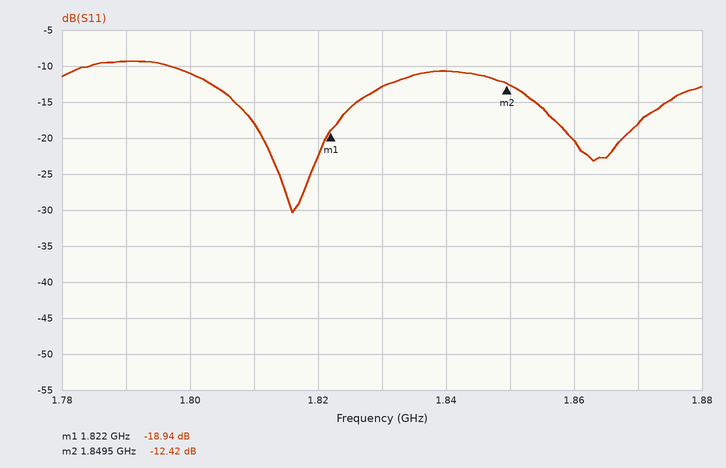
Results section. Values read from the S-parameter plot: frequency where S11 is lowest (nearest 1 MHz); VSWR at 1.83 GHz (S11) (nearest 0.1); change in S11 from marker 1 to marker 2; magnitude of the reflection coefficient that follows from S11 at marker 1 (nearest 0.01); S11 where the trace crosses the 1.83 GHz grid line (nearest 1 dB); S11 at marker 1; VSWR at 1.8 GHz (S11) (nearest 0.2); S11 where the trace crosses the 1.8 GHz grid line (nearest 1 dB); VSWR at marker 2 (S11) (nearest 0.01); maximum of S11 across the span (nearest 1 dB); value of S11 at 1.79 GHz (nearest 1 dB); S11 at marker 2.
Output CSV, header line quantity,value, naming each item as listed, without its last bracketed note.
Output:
quantity,value
frequency where S11 is lowest,1.816 GHz
VSWR at 1.83 GHz (S11),1.6
change in S11 from marker 1 to marker 2,6.52 dB
magnitude of the reflection coefficient that follows from S11 at marker 1,0.11
S11 where the trace crosses the 1.83 GHz grid line,-13 dB
S11 at marker 1,-18.94 dB
VSWR at 1.8 GHz (S11),1.8
S11 where the trace crosses the 1.8 GHz grid line,-11 dB
VSWR at marker 2 (S11),1.63
maximum of S11 across the span,-9 dB
value of S11 at 1.79 GHz,-9 dB
S11 at marker 2,-12.42 dB
